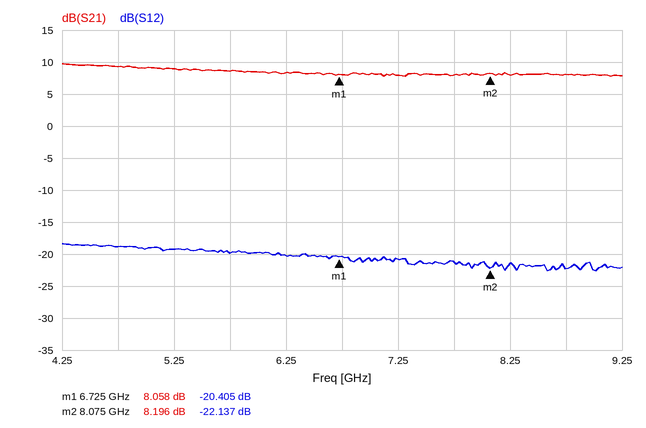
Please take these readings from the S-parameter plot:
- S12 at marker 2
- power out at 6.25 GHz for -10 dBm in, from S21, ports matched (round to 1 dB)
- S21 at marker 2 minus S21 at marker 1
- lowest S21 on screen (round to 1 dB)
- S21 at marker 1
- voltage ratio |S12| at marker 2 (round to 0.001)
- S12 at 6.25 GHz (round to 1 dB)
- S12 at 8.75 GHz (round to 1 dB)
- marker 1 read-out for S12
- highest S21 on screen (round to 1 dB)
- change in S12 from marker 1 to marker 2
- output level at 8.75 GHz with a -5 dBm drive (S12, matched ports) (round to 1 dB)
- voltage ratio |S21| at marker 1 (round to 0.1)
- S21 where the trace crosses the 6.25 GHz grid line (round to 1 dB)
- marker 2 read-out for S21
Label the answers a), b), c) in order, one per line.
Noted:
a) -22.137 dB
b) -2 dBm
c) 0.138 dB
d) 8 dB
e) 8.058 dB
f) 0.078
g) -20 dB
h) -22 dB
i) -20.405 dB
j) 10 dB
k) -1.732 dB
l) -27 dBm
m) 2.5
n) 8 dB
o) 8.196 dB
